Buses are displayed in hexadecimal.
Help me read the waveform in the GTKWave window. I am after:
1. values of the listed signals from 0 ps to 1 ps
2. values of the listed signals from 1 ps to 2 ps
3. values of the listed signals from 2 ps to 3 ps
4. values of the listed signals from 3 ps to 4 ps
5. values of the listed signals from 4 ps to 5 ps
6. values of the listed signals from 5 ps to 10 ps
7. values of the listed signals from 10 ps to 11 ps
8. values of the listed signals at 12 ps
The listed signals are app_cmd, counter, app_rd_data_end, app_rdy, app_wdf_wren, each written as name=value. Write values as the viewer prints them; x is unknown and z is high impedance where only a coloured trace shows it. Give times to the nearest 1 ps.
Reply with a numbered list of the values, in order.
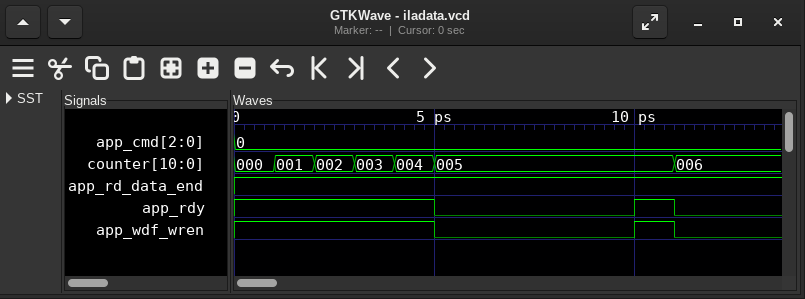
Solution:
1. app_cmd=0, counter=000, app_rd_data_end=1, app_rdy=1, app_wdf_wren=1
2. app_cmd=0, counter=001, app_rd_data_end=1, app_rdy=1, app_wdf_wren=1
3. app_cmd=0, counter=002, app_rd_data_end=1, app_rdy=1, app_wdf_wren=1
4. app_cmd=0, counter=003, app_rd_data_end=1, app_rdy=1, app_wdf_wren=1
5. app_cmd=0, counter=004, app_rd_data_end=1, app_rdy=1, app_wdf_wren=1
6. app_cmd=0, counter=005, app_rd_data_end=1, app_rdy=0, app_wdf_wren=0
7. app_cmd=0, counter=005, app_rd_data_end=1, app_rdy=1, app_wdf_wren=1
8. app_cmd=0, counter=006, app_rd_data_end=1, app_rdy=0, app_wdf_wren=0
